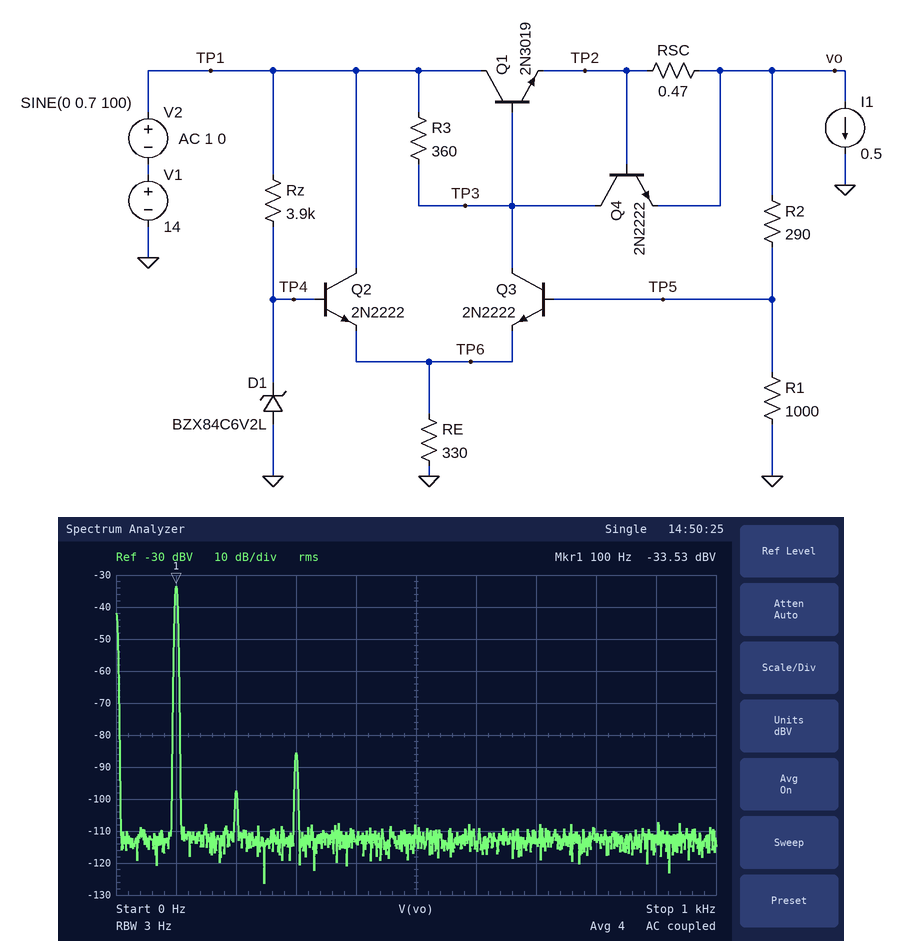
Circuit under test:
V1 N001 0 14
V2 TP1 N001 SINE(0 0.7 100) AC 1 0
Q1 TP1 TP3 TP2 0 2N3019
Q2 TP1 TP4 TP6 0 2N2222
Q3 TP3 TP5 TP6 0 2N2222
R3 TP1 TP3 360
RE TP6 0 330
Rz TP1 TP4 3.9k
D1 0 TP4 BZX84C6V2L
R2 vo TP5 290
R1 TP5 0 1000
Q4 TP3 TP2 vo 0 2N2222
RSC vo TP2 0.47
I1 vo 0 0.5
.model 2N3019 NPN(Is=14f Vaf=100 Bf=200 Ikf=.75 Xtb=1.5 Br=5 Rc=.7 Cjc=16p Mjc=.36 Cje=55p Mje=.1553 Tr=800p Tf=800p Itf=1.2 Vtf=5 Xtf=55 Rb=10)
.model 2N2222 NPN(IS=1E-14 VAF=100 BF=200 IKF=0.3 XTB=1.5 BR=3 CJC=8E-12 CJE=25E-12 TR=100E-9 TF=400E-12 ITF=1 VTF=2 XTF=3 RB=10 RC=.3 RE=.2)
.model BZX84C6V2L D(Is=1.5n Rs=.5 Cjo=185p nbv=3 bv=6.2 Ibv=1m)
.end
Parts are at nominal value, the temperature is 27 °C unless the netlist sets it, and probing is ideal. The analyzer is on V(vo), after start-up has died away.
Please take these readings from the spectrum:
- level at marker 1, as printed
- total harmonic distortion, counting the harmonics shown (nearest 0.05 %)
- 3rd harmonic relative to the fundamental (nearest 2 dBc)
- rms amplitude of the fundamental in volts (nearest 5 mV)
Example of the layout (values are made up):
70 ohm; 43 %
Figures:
-33.53 dBV; 0.25 %; -52 dBc; 20 mV
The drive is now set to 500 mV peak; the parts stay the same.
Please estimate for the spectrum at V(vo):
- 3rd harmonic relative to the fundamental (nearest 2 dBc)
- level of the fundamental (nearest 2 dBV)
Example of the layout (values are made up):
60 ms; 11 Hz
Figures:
-58 dBc; -36 dBV
